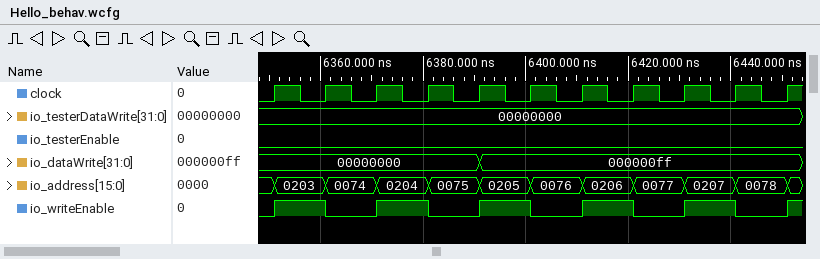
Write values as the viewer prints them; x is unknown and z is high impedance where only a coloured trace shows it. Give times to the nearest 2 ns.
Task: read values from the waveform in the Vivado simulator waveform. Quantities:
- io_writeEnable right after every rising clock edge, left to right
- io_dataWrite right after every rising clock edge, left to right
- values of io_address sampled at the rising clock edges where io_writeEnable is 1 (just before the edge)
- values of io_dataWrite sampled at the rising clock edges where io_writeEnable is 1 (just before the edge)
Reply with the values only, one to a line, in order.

1 0 1 0 1 0 1 0 1 0 1
00000000, 00000000, 00000000, 00000000, 000000ff, 000000ff, 000000ff, 000000ff, 000000ff, 000000ff, 000000ff
0203, 0204, 0205, 0206, 0207
00000000, 00000000, 000000ff, 000000ff, 000000ff
